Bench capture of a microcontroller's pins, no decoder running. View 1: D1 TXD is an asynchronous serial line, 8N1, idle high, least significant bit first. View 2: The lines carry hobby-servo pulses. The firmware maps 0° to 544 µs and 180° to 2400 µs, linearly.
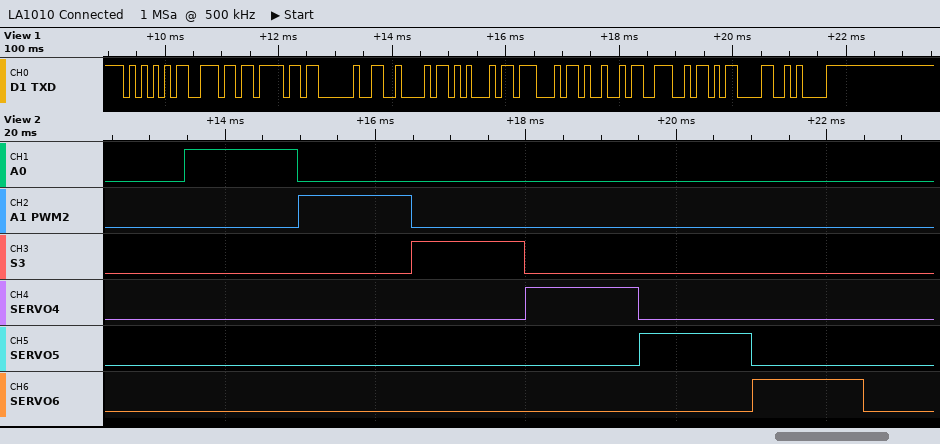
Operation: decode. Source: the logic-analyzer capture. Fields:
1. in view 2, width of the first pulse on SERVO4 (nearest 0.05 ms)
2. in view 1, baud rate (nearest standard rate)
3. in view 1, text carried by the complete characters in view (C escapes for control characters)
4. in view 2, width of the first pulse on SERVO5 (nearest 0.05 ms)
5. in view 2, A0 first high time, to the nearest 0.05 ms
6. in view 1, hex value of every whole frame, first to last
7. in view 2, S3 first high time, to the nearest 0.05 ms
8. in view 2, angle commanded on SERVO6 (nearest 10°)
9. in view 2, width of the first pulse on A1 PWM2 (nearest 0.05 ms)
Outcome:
1.50 ms
9600 baud
"Uno BEGIN\r\n"
1.50 ms
1.50 ms
55 6E 6F 20 42 45 47 49 4E 0D 0A
1.50 ms
90°
1.50 ms
